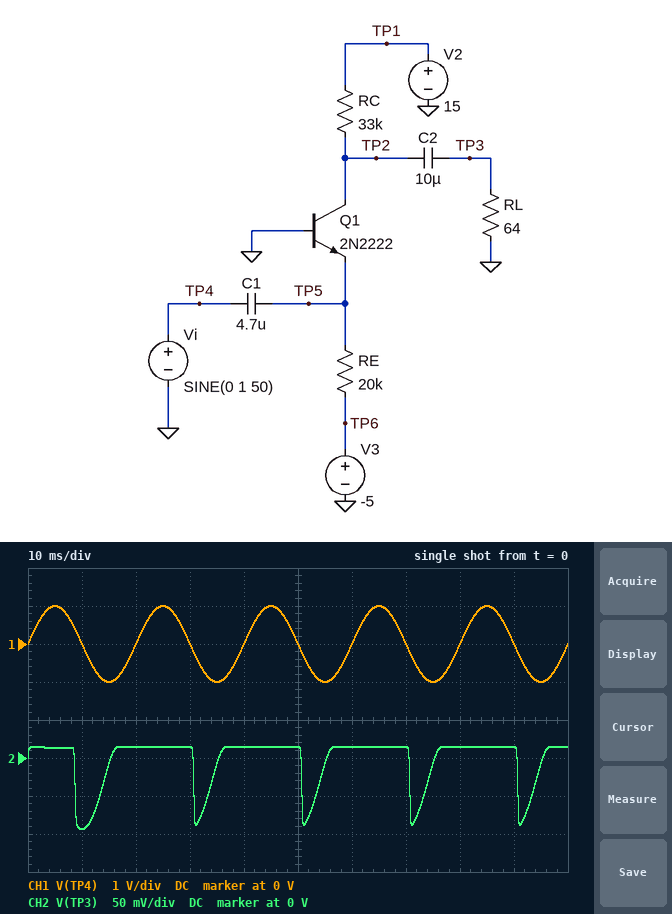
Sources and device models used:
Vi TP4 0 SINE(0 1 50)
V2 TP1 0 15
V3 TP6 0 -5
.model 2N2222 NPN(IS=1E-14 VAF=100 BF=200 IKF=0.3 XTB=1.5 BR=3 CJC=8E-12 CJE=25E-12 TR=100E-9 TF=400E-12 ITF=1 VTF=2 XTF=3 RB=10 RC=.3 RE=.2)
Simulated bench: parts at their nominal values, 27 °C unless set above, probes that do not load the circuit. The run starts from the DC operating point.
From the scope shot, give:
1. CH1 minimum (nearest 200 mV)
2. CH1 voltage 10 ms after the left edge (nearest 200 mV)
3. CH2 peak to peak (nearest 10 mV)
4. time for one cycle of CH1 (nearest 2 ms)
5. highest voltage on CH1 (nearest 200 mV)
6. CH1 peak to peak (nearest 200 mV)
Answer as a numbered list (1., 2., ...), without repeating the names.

1. -1.0 V
2. 0 V
3. 110 mV
4. 20 ms
5. 1.0 V
6. 2.0 V
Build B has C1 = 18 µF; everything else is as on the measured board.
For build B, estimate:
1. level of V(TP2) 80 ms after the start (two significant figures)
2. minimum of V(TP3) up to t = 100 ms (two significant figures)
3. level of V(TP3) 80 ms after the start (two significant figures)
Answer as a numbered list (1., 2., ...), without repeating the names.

1. 6.2 V
2. -360 mV
3. 17 mV
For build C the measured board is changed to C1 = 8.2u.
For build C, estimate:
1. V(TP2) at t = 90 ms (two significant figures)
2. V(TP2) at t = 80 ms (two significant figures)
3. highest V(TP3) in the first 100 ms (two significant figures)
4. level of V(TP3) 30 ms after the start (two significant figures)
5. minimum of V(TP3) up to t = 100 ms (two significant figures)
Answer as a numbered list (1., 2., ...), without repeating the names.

1. 7.2 V
2. 7.0 V
3. 16 mV
4. 15 mV
5. -160 mV
